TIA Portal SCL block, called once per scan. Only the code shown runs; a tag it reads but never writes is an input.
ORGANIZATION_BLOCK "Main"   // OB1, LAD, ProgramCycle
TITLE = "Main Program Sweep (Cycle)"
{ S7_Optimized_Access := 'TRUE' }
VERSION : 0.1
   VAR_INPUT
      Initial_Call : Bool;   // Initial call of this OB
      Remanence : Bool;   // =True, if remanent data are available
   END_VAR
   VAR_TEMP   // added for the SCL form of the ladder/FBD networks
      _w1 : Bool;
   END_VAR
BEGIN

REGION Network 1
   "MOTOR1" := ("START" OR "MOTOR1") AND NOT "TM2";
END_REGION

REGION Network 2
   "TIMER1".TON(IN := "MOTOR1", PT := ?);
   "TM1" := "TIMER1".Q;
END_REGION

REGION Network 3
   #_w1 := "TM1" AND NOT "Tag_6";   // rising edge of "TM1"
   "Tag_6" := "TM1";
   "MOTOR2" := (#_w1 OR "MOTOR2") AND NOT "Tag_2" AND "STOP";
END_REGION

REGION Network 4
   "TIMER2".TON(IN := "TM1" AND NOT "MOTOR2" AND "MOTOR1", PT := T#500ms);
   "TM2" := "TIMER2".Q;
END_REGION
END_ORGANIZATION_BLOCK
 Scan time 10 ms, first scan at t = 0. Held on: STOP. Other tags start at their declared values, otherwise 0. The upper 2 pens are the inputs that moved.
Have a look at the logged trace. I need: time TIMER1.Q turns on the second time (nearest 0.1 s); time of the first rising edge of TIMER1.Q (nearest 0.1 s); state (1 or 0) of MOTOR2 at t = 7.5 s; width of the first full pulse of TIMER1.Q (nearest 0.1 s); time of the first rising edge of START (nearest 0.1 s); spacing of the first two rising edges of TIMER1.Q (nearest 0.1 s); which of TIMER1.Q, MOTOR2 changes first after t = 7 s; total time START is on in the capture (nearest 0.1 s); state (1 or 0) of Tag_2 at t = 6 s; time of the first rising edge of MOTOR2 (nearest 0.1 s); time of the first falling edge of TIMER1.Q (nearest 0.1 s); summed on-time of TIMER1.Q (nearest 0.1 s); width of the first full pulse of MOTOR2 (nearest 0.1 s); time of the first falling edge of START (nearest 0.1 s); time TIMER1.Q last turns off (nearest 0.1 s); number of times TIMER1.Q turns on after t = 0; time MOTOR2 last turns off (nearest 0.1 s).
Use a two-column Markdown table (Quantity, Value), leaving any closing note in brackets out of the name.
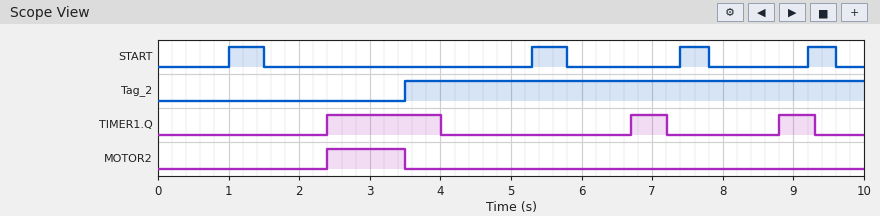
| Quantity | Value |
|---|---|
| time TIMER1.Q turns on the second time | 6.7 s |
| time of the first rising edge of TIMER1.Q | 2.4 s |
| state (1 or 0) of MOTOR2 at t = 7.5 s | 0 |
| width of the first full pulse of TIMER1.Q | 1.6 s |
| time of the first rising edge of START | 1.0 s |
| spacing of the first two rising edges of TIMER1.Q | 4.3 s |
| which of TIMER1.Q, MOTOR2 changes first after t = 7 s | TIMER1.Q |
| total time START is on in the capture | 1.8 s |
| state (1 or 0) of Tag_2 at t = 6 s | 1 |
| time of the first rising edge of MOTOR2 | 2.4 s |
| time of the first falling edge of TIMER1.Q | 4.0 s |
| summed on-time of TIMER1.Q | 2.6 s |
| width of the first full pulse of MOTOR2 | 1.1 s |
| time of the first falling edge of START | 1.5 s |
| time TIMER1.Q last turns off | 9.3 s |
| number of times TIMER1.Q turns on after t = 0 | 3 |
| time MOTOR2 last turns off | 3.5 s |
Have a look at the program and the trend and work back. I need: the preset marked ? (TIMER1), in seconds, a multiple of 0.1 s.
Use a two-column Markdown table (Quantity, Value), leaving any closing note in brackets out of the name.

| Quantity | Value |
|---|---|
| the preset marked ? (TIMER1), in seconds, a multiple of 0.1 s | 1.4 s |
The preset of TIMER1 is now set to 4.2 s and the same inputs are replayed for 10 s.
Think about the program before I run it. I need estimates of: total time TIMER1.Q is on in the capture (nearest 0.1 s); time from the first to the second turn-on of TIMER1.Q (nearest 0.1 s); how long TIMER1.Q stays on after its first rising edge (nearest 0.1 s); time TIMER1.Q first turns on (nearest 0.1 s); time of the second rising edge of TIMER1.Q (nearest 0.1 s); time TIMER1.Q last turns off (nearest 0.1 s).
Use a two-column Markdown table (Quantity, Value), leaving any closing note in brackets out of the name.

| Quantity | Value |
|---|---|
| total time TIMER1.Q is on in the capture | 0.6 s |
| time from the first to the second turn-on of TIMER1.Q | 4.7 s |
| how long TIMER1.Q stays on after its first rising edge | 0.5 s |
| time TIMER1.Q first turns on | 5.2 s |
| time of the second rising edge of TIMER1.Q | 9.9 s |
| time TIMER1.Q last turns off | 5.7 s |
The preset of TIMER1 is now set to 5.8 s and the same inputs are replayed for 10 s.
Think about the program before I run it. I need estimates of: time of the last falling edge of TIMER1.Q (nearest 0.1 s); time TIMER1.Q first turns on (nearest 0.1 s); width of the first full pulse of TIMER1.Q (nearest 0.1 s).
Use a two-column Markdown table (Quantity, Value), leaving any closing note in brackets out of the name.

| Quantity | Value |
|---|---|
| time of the last falling edge of TIMER1.Q | 7.3 s |
| time TIMER1.Q first turns on | 6.8 s |
| width of the first full pulse of TIMER1.Q | 0.5 s |
